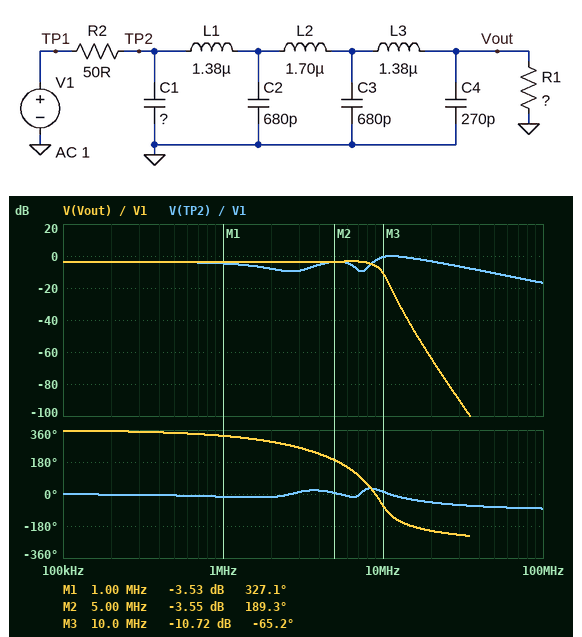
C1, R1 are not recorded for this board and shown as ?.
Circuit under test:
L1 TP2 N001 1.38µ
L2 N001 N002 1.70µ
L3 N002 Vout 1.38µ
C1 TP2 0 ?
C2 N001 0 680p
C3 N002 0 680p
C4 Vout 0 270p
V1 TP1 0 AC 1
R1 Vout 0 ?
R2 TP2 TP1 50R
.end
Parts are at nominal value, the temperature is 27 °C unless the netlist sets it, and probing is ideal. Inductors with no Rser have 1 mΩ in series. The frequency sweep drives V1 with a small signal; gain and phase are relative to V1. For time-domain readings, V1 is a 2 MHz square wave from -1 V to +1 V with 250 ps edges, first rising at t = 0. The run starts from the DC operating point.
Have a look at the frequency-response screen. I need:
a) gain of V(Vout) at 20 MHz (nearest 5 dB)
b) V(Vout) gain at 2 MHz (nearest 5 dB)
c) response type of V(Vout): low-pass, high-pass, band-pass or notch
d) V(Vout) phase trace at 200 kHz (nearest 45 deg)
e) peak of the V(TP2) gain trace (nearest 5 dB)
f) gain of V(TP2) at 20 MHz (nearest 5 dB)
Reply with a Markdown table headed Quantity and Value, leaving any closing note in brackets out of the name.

| Quantity | Value |
|---|---|
| gain of V(Vout) at 20 MHz | -65 dB |
| V(Vout) gain at 2 MHz | -5 dB |
| response type of V(Vout): low-pass, high-pass, band-pass or notch | low-pass |
| V(Vout) phase trace at 200 kHz | 360 deg |
| peak of the V(TP2) gain trace | 0 dB |
| gain of V(TP2) at 20 MHz | -5 dB |
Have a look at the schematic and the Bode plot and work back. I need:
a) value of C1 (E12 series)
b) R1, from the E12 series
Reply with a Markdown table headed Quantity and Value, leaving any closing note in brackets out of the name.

| Quantity | Value |
|---|---|
| value of C1 | 220 pF |
| R1, from the E12 series | 100 Ω |
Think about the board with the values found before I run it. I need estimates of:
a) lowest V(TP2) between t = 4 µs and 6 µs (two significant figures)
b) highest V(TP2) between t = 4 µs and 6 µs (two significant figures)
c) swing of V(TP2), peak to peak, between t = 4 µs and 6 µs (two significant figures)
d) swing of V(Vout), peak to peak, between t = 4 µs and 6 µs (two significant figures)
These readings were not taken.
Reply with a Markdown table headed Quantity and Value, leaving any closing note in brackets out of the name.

| Quantity | Value |
|---|---|
| lowest V(TP2) between t = 4 µs and 6 µs | -710 mV |
| highest V(TP2) between t = 4 µs and 6 µs | 710 mV |
| swing of V(TP2), peak to peak, between t = 4 µs and 6 µs | 1.4 V |
| swing of V(Vout), peak to peak, between t = 4 µs and 6 µs | 1.8 V |
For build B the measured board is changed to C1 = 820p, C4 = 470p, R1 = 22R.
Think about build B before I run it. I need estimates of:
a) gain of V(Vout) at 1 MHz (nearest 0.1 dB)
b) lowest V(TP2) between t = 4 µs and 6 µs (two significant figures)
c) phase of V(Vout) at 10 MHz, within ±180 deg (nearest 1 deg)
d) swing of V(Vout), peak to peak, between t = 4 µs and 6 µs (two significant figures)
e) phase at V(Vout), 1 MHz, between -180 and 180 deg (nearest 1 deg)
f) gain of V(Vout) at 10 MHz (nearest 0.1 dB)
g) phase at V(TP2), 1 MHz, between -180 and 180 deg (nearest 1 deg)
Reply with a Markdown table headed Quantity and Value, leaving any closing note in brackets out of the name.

| Quantity | Value |
|---|---|
| gain of V(Vout) at 1 MHz | -10.0 dB |
| lowest V(TP2) between t = 4 µs and 6 µs | -770 mV |
| phase of V(Vout) at 10 MHz, within ±180 deg | -161 deg |
| swing of V(Vout), peak to peak, between t = 4 µs and 6 µs | 790 mV |
| phase at V(Vout), 1 MHz, between -180 and 180 deg | -38 deg |
| gain of V(Vout) at 10 MHz | -28.9 dB |
| phase at V(TP2), 1 MHz, between -180 and 180 deg | 18 deg |
